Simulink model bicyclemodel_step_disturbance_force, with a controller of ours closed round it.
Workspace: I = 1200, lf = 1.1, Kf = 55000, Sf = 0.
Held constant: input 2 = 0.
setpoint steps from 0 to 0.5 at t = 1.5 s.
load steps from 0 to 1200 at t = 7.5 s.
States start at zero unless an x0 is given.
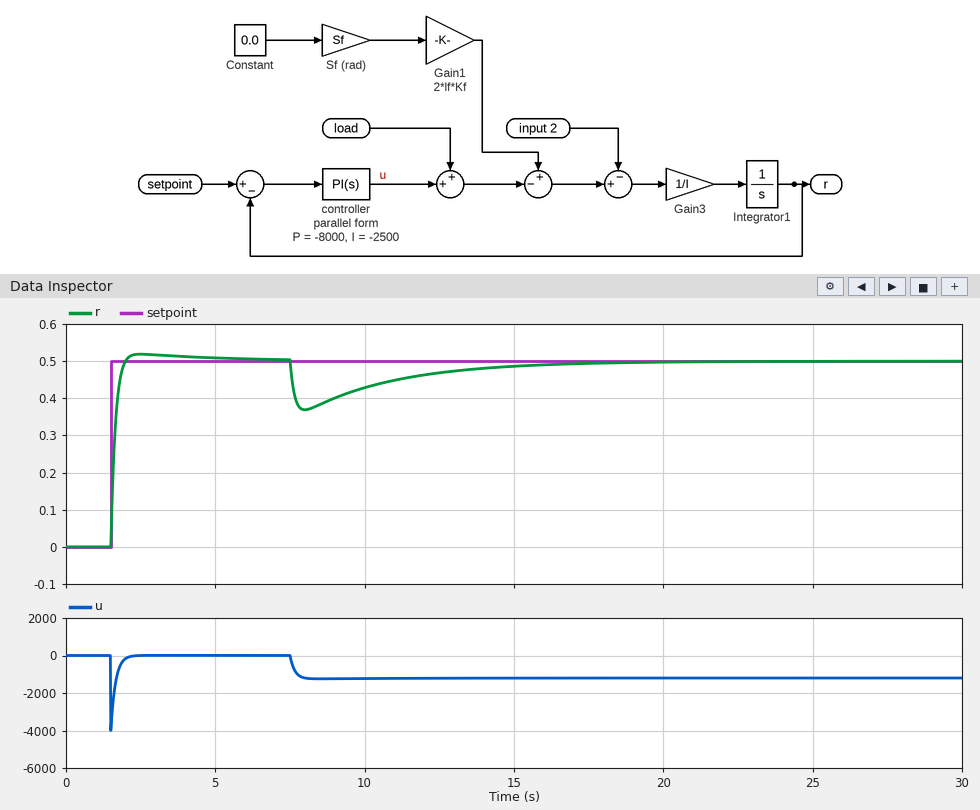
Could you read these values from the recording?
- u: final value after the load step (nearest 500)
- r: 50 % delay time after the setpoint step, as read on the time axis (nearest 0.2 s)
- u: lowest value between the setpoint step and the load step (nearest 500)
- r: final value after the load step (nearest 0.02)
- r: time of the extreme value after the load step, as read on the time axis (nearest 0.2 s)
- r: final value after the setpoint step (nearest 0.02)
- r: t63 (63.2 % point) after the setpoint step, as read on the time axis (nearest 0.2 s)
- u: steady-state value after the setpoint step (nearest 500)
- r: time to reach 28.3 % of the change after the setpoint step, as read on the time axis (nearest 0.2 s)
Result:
-1000
1.6 s
-4000
0.50
8.0 s
0.50
1.6 s
0
1.6 s
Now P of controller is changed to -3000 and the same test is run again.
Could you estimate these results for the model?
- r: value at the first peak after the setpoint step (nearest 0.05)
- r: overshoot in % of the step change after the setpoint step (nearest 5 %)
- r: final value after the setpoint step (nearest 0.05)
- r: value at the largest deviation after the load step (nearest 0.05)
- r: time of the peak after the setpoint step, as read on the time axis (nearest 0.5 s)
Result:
0.60
15 %
0.50
0.20
3.0 s
